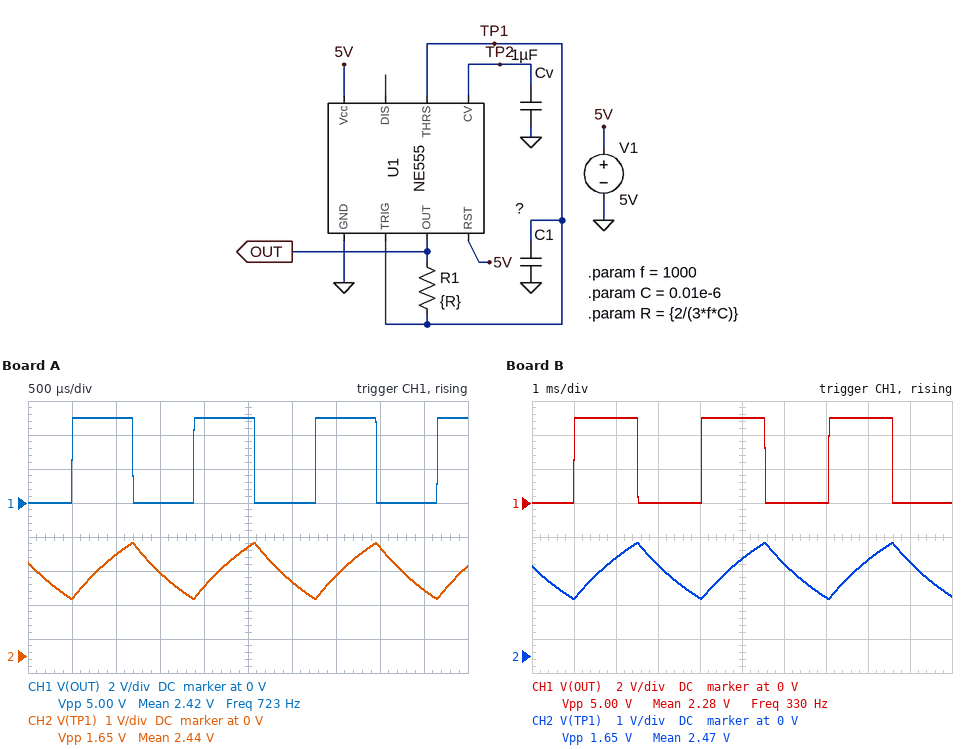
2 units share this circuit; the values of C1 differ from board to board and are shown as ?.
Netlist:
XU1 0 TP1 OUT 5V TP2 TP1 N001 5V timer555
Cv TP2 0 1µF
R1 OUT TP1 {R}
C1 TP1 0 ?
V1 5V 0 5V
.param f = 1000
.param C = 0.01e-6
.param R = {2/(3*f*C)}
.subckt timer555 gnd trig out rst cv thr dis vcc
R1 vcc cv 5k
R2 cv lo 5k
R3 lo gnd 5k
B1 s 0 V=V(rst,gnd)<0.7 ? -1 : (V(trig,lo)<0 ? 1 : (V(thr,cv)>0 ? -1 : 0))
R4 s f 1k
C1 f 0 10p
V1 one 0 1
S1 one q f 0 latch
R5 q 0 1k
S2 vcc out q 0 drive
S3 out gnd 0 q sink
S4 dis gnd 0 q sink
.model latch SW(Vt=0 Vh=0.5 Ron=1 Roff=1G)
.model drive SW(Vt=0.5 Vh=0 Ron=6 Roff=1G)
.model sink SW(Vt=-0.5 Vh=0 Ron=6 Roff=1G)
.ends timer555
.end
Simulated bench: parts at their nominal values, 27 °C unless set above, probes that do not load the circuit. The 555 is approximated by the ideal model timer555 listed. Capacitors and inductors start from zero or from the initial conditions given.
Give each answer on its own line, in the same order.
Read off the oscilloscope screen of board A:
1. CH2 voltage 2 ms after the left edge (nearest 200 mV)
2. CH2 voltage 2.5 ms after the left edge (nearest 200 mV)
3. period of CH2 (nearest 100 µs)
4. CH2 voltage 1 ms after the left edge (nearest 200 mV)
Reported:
2.0 V
3.2 V
1.4 ms
3.0 V
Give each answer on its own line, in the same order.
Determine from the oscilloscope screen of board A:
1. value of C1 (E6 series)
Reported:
15 nF
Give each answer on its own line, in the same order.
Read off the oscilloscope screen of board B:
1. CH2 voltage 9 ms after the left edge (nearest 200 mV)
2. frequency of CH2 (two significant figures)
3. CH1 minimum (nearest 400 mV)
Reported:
2.8 V
330 Hz
0 V
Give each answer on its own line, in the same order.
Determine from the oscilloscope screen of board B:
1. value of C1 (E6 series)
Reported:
33 nF
